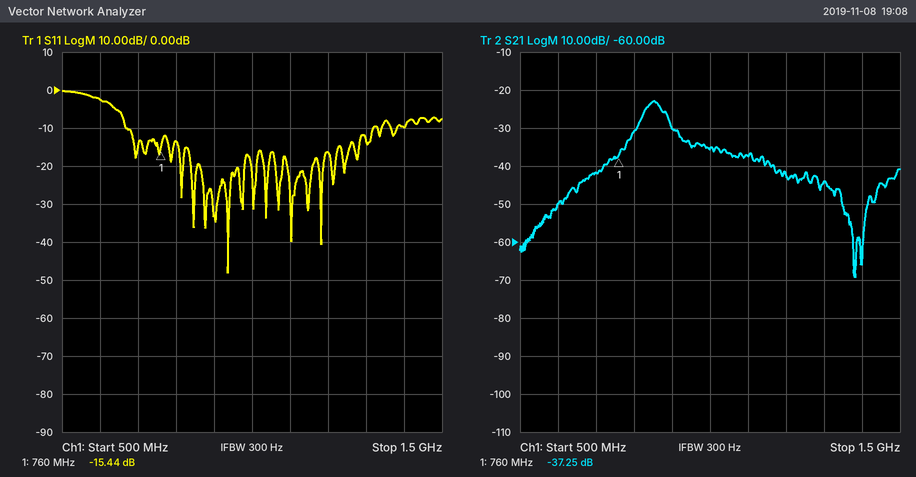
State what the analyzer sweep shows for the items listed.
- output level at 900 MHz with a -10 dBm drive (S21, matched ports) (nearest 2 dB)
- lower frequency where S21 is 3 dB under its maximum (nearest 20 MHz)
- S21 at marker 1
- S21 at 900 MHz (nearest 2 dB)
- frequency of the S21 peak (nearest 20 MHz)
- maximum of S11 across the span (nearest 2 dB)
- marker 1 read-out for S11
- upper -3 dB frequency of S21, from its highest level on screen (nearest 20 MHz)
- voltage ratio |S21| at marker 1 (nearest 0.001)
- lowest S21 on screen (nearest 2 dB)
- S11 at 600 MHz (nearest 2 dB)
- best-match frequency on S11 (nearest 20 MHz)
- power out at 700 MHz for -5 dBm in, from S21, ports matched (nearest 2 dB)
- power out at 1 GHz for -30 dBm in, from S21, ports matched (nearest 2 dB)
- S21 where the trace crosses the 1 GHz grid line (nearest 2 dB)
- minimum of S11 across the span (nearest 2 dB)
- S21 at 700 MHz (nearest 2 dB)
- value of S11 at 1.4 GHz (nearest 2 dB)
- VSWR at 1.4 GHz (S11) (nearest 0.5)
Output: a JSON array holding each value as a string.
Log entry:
["-40 dBm", "820 MHz", "-37.25 dB", "-30 dB", "860 MHz", "0 dB", "-15.44 dB", "880 MHz", "0.014", "-70 dB", "-2 dB", "940 MHz", "-46 dBm", "-66 dBm", "-36 dB", "-48 dB", "-42 dB", "-10 dB", "2.0"]
